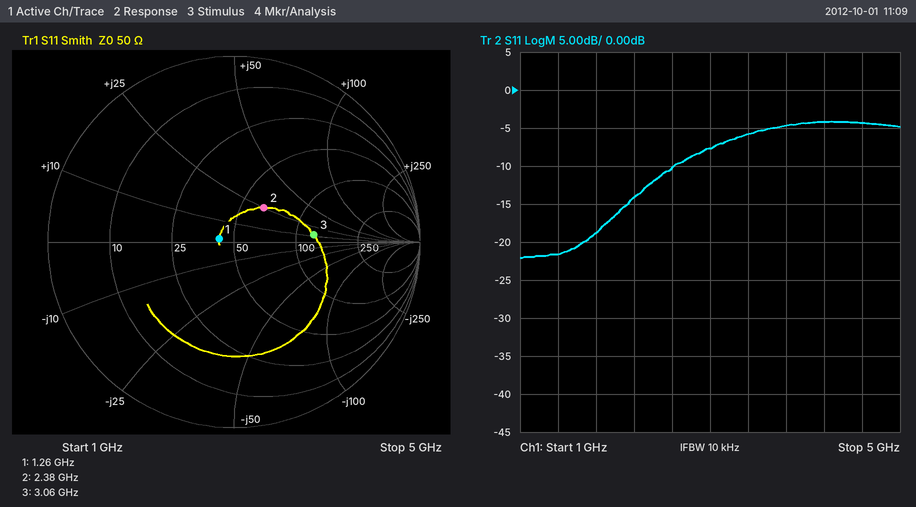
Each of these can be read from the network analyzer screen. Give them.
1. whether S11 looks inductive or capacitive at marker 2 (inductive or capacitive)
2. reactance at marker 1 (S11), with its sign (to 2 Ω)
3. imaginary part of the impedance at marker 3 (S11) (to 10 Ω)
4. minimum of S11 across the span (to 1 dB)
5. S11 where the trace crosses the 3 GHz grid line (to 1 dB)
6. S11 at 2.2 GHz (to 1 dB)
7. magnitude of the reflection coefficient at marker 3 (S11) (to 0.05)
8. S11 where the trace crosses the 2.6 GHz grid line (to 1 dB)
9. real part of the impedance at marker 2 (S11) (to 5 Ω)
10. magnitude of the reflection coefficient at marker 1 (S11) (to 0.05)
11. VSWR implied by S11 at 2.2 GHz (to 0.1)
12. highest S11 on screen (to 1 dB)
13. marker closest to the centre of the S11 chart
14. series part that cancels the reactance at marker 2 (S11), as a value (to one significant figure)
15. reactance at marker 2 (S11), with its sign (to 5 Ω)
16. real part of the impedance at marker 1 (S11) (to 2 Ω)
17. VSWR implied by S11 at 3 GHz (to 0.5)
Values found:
inductive
+2 Ω
+10 Ω
-22 dB
-8 dB
-14 dB
0.45
-10 dB
65 Ω
0.10
1.5
-4 dB
marker 1
3 pF
+25 Ω
42 Ω
2.5
